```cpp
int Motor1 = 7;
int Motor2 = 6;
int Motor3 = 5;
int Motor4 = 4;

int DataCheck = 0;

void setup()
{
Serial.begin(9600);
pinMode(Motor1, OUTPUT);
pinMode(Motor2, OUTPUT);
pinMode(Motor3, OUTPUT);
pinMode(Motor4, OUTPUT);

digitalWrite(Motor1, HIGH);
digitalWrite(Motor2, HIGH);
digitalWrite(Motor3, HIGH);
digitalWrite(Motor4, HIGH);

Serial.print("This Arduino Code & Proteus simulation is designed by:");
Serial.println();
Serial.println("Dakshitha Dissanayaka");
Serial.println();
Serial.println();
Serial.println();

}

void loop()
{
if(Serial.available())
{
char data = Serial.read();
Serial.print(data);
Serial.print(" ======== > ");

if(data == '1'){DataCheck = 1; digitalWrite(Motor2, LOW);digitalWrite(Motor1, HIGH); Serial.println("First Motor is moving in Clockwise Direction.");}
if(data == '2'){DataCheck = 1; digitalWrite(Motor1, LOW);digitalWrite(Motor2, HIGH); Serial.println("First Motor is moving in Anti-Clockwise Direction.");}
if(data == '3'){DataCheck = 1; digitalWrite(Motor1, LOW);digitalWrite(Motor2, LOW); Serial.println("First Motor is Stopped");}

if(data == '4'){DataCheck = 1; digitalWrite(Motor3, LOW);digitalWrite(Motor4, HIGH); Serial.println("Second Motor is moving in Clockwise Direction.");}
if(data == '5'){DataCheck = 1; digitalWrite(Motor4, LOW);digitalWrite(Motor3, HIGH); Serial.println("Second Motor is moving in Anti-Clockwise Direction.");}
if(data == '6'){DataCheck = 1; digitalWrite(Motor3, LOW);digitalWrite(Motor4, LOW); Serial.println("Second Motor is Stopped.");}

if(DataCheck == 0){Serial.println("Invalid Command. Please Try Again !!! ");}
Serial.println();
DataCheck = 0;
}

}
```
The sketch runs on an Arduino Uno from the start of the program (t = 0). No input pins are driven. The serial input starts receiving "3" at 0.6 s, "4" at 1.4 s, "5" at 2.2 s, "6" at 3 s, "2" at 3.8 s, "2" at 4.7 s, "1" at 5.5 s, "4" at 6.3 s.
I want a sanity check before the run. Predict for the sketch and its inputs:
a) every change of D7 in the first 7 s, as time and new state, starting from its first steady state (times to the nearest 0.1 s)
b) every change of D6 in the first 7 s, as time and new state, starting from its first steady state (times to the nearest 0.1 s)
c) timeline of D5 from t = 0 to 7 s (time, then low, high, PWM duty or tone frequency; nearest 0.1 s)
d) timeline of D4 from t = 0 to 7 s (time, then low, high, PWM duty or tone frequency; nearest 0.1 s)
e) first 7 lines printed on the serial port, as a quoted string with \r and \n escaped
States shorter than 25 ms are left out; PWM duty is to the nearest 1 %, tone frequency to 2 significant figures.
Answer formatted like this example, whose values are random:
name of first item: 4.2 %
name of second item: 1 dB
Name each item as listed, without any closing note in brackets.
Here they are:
every change of D7 in the first 7 s, as time and new state, starting from its first steady state: 0 s high; 0.6 s low; 5.5 s high
every change of D6 in the first 7 s, as time and new state, starting from its first steady state: 0 s high; 0.6 s low; 3.8 s high; 5.5 s low
timeline of D5 from t = 0 to 7 s: 0 s high; 1.4 s low; 2.2 s high; 3 s low
timeline of D4 from t = 0 to 7 s: 0 s high; 2.2 s low; 6.3 s high
first 7 lines printed on the serial port, as a quoted string with \r and \n escaped: "This Arduino Code & Proteus simulation is designed by:\r\nDakshitha Dissanayaka\r\n\r\n\r\n\r\n3 ======== > First Motor is Stopped\r\n\r\n"
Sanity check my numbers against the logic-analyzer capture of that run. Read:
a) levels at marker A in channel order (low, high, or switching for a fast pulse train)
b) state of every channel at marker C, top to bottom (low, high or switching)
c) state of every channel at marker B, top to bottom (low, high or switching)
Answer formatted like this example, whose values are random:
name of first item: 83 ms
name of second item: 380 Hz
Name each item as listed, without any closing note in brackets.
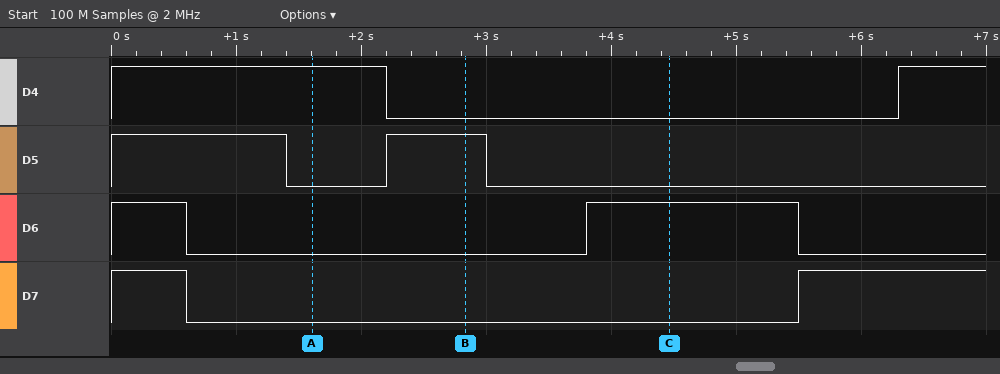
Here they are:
levels at marker A in channel order: D4 high, D5 low, D6 low, D7 low
state of every channel at marker C, top to bottom: D4 low, D5 low, D6 high, D7 low
state of every channel at marker B, top to bottom: D4 low, D5 high, D6 low, D7 low
